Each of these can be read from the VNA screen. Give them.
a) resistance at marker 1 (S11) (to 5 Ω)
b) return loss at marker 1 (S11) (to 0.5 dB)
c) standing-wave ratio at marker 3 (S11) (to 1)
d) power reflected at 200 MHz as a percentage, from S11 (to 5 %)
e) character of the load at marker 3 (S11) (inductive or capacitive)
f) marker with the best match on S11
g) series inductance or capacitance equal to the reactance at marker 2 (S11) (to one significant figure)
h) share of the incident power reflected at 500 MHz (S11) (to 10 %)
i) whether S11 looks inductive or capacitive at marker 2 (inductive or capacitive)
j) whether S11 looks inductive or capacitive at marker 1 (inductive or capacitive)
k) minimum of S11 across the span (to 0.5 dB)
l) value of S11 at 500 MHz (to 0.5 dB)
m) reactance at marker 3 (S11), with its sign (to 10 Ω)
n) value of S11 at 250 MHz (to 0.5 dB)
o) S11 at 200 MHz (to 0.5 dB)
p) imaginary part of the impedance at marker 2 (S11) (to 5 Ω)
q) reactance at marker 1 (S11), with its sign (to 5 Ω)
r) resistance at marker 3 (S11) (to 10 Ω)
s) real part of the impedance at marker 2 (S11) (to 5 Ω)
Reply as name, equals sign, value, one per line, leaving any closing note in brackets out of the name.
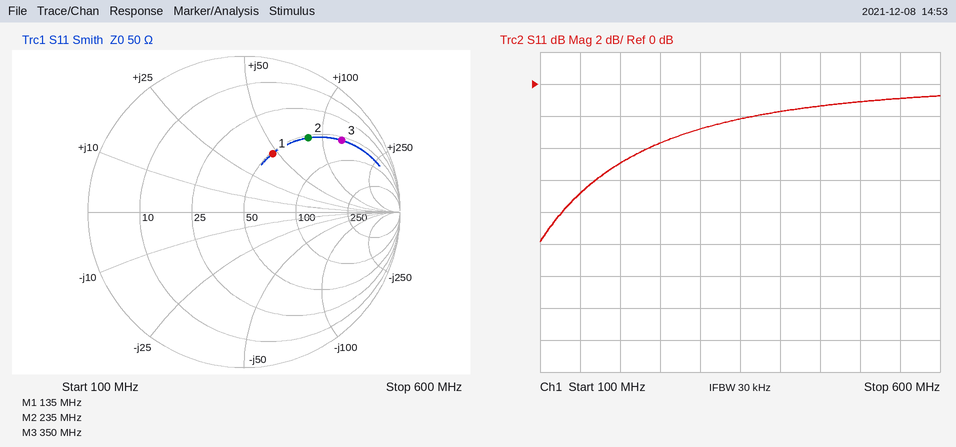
resistance at marker 1 (S11) = 50 Ω
return loss at marker 1 (S11) = 7.5 dB
standing-wave ratio at marker 3 (S11) = 8
power reflected at 200 MHz as a percentage, from S11 = 30 %
character of the load at marker 3 (S11) = inductive
marker with the best match on S11 = marker 1
series inductance or capacitance equal to the reactance at marker 2 (S11) = 60 nH
share of the incident power reflected at 500 MHz (S11) = 80 %
whether S11 looks inductive or capacitive at marker 2 = inductive
whether S11 looks inductive or capacitive at marker 1 = inductive
minimum of S11 across the span = -10.0 dB
value of S11 at 500 MHz = -1.0 dB
reactance at marker 3 (S11), with its sign = +130 Ω
value of S11 at 250 MHz = -3.5 dB
S11 at 200 MHz = -5.0 dB
imaginary part of the impedance at marker 2 (S11) = +85 Ω
reactance at marker 1 (S11), with its sign = +45 Ω
resistance at marker 3 (S11) = 60 Ω
real part of the impedance at marker 2 (S11) = 55 Ω
